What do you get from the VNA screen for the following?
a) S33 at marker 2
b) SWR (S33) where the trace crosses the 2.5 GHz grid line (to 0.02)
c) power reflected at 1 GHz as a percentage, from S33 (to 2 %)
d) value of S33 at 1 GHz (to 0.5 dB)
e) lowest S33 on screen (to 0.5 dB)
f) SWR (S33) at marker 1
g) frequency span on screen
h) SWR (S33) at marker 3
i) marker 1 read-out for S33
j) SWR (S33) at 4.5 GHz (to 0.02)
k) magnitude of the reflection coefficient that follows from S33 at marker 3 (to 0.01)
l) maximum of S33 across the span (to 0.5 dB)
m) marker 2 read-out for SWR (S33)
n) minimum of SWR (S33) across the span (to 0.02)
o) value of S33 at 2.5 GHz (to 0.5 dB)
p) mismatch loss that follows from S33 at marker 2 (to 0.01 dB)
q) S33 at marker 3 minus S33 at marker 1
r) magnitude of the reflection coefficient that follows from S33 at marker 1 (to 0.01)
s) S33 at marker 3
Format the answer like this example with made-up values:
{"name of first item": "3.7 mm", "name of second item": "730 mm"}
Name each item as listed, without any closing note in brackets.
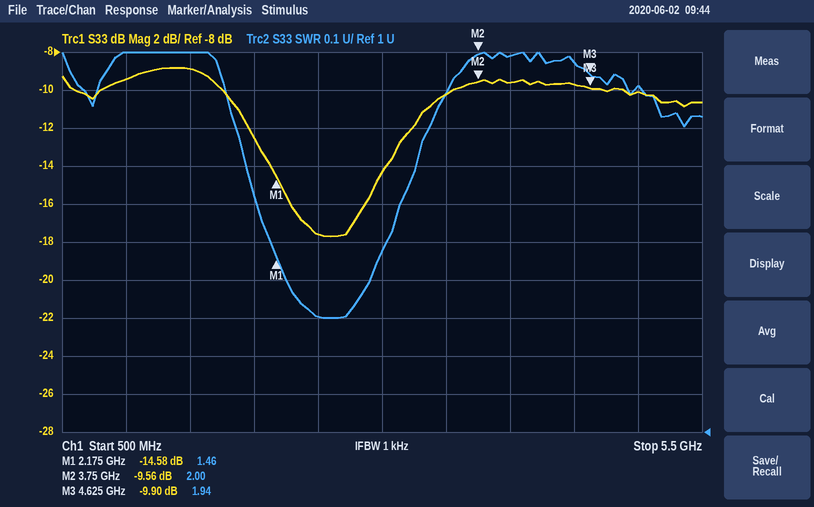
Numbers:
{"S33 at marker 2": "-9.56 dB", "SWR (S33) where the trace crosses the 2.5 GHz grid line": "1.30", "power reflected at 1 GHz as a percentage, from S33": "12 %", "value of S33 at 1 GHz": "-9.5 dB", "lowest S33 on screen": "-17.5 dB", "SWR (S33) at marker 1": "1.46", "frequency span on screen": "5 GHz", "SWR (S33) at marker 3": "1.94", "marker 1 read-out for S33": "-14.58 dB", "SWR (S33) at 4.5 GHz": "1.98", "magnitude of the reflection coefficient that follows from S33 at marker 3": "0.32", "maximum of S33 across the span": "-9.0 dB", "marker 2 read-out for SWR": "2.00", "minimum of SWR (S33) across the span": "1.30", "value of S33 at 2.5 GHz": "-17.5 dB", "mismatch loss that follows from S33 at marker 2": "0.51 dB", "S33 at marker 3 minus S33 at marker 1": "4.68 dB", "magnitude of the reflection coefficient that follows from S33 at marker 1": "0.19", "S33 at marker 3": "-9.90 dB"}
